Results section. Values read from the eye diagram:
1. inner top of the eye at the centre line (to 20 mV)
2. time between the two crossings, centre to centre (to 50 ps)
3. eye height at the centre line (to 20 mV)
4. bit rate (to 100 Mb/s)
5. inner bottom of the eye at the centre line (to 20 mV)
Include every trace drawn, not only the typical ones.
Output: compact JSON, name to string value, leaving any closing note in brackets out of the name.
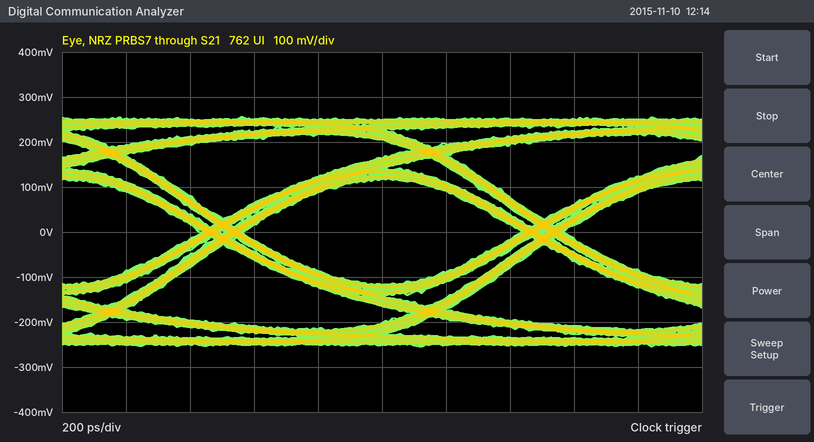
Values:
{"inner top of the eye at the centre line": "120 mV", "time between the two crossings, centre to centre": "1.00 ns", "eye height at the centre line": "240 mV", "bit rate": "1.0 Gb/s", "inner bottom of the eye at the centre line": "-120 mV"}
